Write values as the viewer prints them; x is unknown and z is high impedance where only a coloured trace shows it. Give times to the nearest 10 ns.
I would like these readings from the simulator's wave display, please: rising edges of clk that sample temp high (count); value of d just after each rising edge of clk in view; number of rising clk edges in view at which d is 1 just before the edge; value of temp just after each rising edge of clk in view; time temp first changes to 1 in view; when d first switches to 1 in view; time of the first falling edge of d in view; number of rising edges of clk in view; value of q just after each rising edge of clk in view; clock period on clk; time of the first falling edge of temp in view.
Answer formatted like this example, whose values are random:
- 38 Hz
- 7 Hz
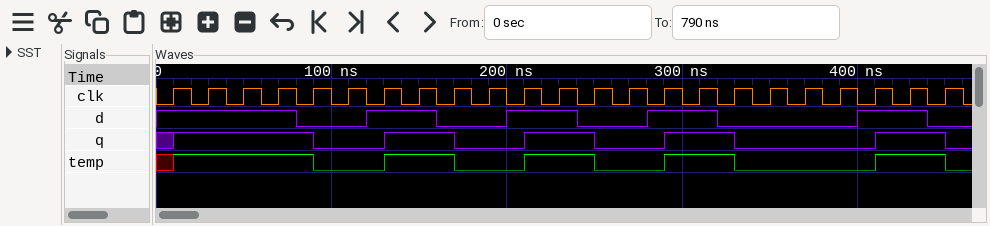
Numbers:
- 12
- 1 1 1 1 0 0 1 1 0 0 1 1 0 0 1 1 0 0 0 0 1 1 0
- 12
- 1 1 1 1 0 0 1 1 0 0 1 1 0 0 1 1 0 0 0 0 1 1 0
- 10 ns
- 120 ns
- 80 ns
- 23
- 1 1 1 1 0 0 1 1 0 0 1 1 0 0 1 1 0 0 0 0 1 1 0
- 20 ns
- 90 ns
